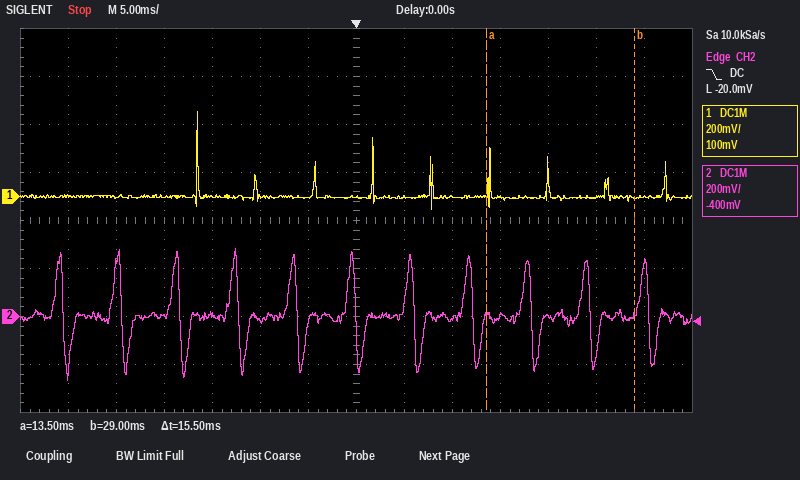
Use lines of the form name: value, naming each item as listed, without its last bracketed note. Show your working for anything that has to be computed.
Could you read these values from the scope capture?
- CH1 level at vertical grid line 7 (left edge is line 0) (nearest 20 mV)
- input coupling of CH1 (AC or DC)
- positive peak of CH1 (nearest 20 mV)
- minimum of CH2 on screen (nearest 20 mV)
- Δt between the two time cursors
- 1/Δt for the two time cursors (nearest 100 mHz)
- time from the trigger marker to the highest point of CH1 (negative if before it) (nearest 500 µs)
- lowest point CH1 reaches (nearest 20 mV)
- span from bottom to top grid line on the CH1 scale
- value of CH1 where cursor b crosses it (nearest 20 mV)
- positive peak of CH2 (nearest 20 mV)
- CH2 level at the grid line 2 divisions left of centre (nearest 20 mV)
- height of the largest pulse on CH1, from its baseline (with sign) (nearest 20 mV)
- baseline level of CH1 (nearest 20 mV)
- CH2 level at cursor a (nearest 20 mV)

CH1 level at vertical grid line 7 (left edge is line 0): 0 mV
input coupling of CH1: DC
positive peak of CH1: 360 mV
minimum of CH2 on screen: -260 mV
Δt between the two time cursors: 15.5 ms
1/Δt for the two time cursors: 1 / 15.5 ms ≈ 64.5 Hz
time from the trigger marker to the highest point of CH1 (negative if before it): -16.5 ms
lowest point CH1 reaches: -60 mV
span from bottom to top grid line on the CH1 scale: 1.6 V
value of CH1 where cursor b crosses it: 0 mV
positive peak of CH2: 280 mV
CH2 level at the grid line 2 divisions left of centre: -20 mV
height of the largest pulse on CH1, from its baseline (with sign): 360 mV − (0 mV) = +360 mV
baseline level of CH1: 0 mV
CH2 level at cursor a: 0 mV
